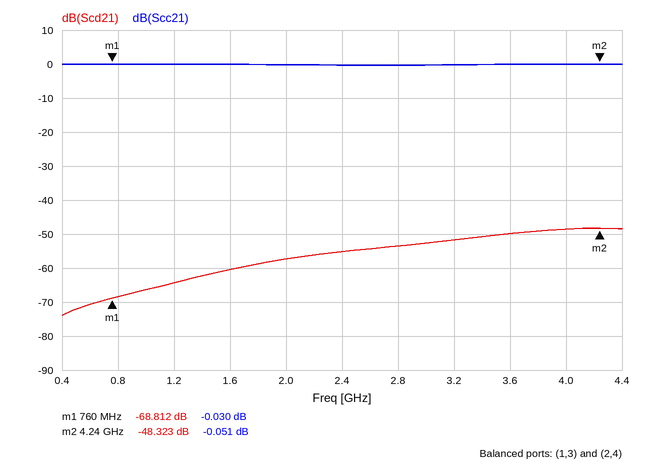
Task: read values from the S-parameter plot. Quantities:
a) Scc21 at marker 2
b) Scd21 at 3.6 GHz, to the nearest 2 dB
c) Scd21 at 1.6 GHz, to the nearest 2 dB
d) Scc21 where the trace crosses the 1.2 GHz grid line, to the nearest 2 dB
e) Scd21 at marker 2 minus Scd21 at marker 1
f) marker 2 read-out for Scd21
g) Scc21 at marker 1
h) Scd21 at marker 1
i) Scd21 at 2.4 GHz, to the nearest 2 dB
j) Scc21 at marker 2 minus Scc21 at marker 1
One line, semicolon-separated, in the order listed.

-0.051 dB; -50 dB; -60 dB; 0 dB; 20.489 dB; -48.323 dB; -0.030 dB; -68.812 dB; -56 dB; -0.021 dB
